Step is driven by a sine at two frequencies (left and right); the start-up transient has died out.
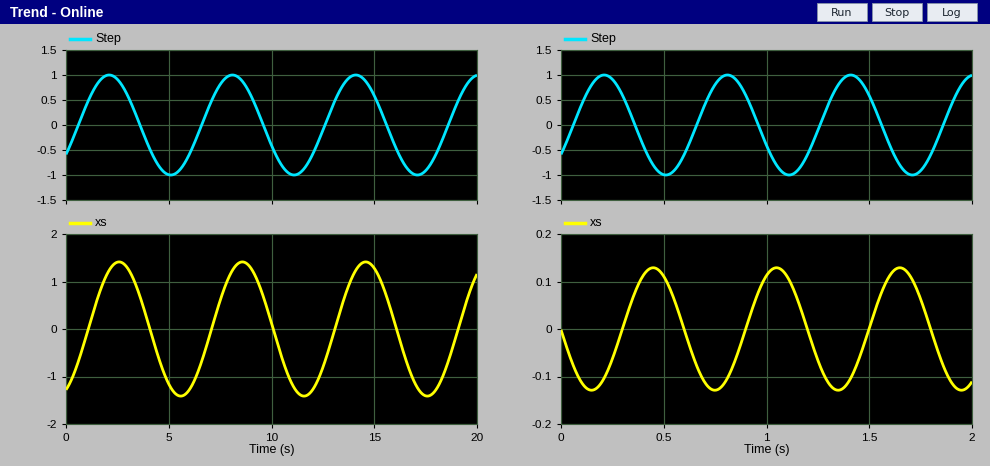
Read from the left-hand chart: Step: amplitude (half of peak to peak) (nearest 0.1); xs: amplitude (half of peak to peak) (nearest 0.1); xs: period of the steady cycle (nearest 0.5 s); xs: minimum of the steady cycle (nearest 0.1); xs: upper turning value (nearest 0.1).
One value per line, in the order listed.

1.0
1.4
6.0 s
-1.4
1.4
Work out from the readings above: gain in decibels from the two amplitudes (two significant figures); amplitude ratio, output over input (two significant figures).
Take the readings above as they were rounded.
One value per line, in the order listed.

2.9 dB
1.4
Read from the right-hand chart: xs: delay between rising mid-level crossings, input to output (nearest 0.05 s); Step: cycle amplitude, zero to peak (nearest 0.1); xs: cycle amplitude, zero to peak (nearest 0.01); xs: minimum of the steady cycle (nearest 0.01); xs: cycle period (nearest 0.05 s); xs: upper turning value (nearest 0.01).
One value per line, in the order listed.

0.25 s
1.0
0.13
-0.13
0.60 s
0.13
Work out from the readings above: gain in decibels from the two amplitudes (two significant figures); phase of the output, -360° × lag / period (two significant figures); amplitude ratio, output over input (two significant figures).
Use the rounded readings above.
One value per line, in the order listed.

-18 dB
-150°
0.13
